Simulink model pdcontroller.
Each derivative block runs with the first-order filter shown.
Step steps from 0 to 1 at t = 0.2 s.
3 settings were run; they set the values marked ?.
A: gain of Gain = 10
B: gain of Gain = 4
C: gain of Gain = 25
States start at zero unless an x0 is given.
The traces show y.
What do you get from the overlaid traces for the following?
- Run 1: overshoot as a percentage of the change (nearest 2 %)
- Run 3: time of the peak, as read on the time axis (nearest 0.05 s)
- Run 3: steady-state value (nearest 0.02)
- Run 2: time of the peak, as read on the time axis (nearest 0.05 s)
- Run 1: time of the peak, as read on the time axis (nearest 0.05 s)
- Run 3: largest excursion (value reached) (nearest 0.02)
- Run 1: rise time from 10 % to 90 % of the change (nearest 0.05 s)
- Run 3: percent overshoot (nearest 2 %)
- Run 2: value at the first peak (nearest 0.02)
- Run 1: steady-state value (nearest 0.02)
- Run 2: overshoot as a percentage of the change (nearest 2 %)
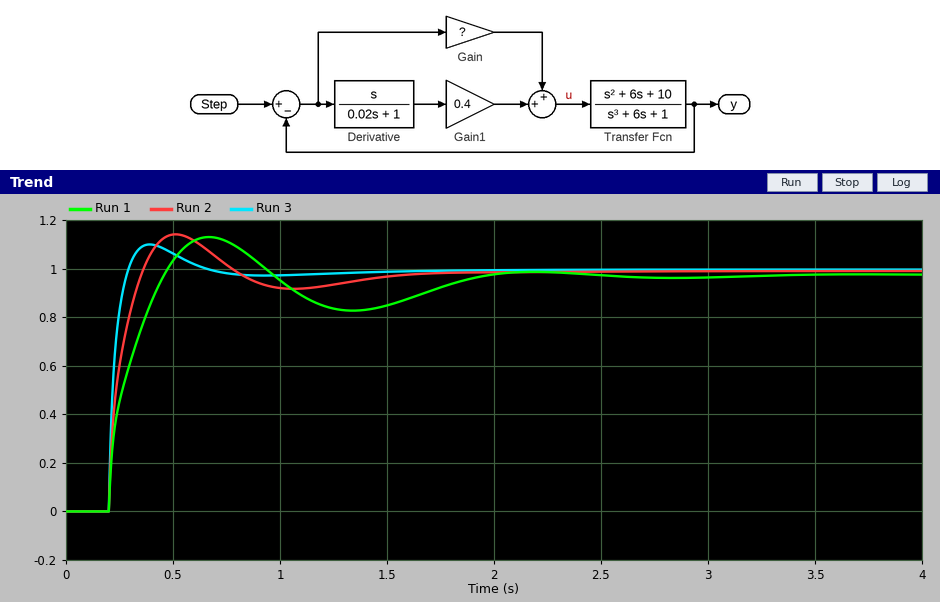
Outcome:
16 %
0.40 s
1.00
0.50 s
0.65 s
1.10
0.20 s
10 %
1.14
0.98
16 %
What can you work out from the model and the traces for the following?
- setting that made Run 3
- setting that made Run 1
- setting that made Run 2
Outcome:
C
B
A
